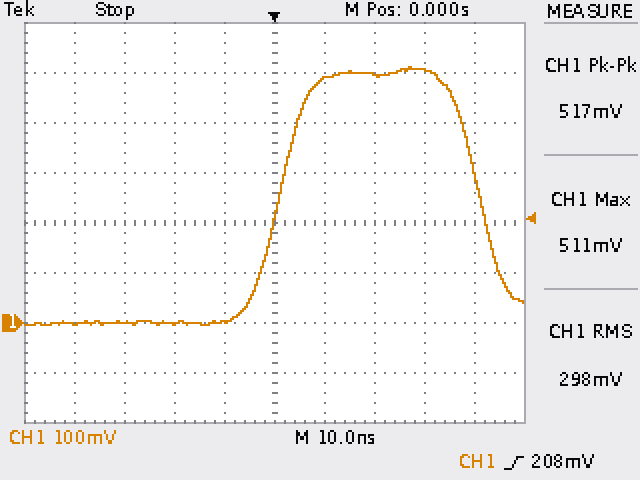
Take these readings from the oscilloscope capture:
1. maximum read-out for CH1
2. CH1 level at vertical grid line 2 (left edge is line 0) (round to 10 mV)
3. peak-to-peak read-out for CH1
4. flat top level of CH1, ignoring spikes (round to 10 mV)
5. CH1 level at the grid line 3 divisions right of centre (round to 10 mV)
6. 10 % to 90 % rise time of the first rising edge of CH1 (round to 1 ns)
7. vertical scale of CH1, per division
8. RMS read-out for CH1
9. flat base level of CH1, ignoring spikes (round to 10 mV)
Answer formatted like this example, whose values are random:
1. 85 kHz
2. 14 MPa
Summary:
1. 511 mV
2. 0 mV
3. 517 mV
4. 500 mV
5. 510 mV
6. 11 ns
7. 100 mV
8. 298 mV
9. 0 mV
